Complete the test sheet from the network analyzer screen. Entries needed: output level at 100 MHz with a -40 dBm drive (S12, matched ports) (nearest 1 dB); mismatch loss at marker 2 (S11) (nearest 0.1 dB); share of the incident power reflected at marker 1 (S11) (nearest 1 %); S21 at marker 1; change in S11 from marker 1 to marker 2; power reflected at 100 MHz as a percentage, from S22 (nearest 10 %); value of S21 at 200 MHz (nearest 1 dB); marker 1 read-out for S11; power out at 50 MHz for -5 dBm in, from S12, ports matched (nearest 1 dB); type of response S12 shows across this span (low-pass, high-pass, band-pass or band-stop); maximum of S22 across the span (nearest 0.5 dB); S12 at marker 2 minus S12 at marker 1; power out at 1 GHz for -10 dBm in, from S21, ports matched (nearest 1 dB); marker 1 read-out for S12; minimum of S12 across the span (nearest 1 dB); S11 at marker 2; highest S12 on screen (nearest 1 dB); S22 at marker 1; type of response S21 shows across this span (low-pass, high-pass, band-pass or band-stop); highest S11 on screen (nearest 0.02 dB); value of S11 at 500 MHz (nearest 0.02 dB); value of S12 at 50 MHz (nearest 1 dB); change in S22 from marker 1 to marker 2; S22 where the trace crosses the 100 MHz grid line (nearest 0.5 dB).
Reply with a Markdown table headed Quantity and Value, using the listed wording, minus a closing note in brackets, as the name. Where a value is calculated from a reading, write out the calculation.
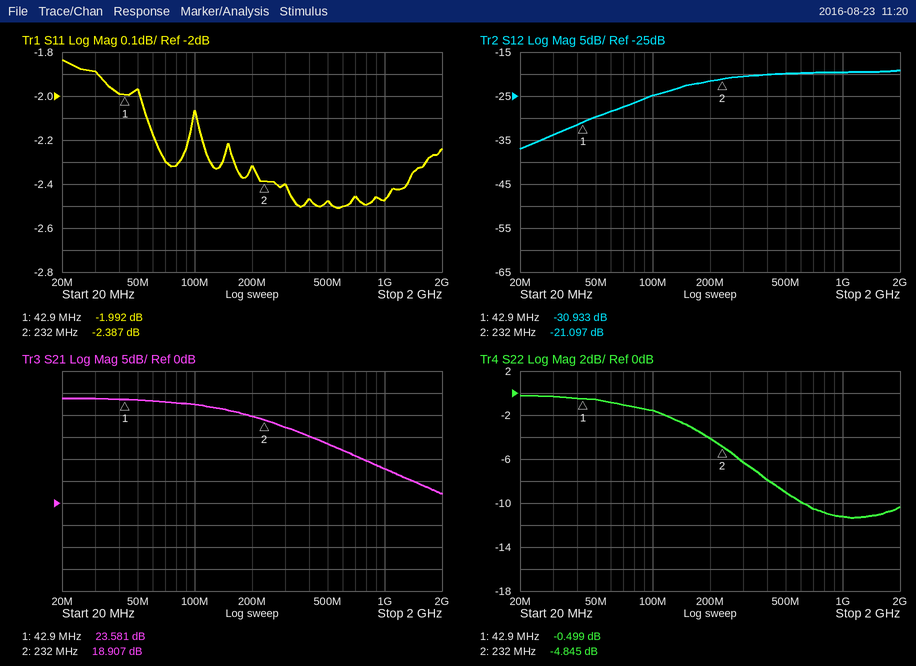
| Quantity | Value |
|---|---|
| output level at 100 MHz with a -40 dBm drive (S12, matched ports) | -40 dBm + (-25 dB) = -65 dBm |
| mismatch loss at marker 2 (S11) | −10 log10(1 − 10^(-2.387/10)) ≈ 3.7 dB |
| share of the incident power reflected at marker 1 (S11) | 10^(-1.992/10) ≈ 63 % |
| S21 at marker 1 | 23.581 dB |
| change in S11 from marker 1 to marker 2 | -2.387 − (-1.992) = -0.395 dB |
| power reflected at 100 MHz as a percentage, from S22 | 10^(-1.5/10) ≈ 70.8 %, so 70 % to the nearest 10 % |
| value of S21 at 200 MHz | 20 dB |
| marker 1 read-out for S11 | -1.992 dB |
| power out at 50 MHz for -5 dBm in, from S12, ports matched | -5 dBm + (-30 dB) = -35 dBm |
| type of response S12 shows across this span | high-pass |
| maximum of S22 across the span | 0.0 dB |
| S12 at marker 2 minus S12 at marker 1 | -21.097 − (-30.933) = 9.836 dB |
| power out at 1 GHz for -10 dBm in, from S21, ports matched | -10 dBm + (8 dB) = -2 dBm |
| marker 1 read-out for S12 | -30.933 dB |
| minimum of S12 across the span | -37 dB |
| S11 at marker 2 | -2.387 dB |
| highest S12 on screen | -19 dB |
| S22 at marker 1 | -0.499 dB |
| type of response S21 shows across this span | low-pass |
| highest S11 on screen | -1.84 dB |
| value of S11 at 500 MHz | -2.48 dB |
| value of S12 at 50 MHz | -30 dB |
| change in S22 from marker 1 to marker 2 | -4.845 − (-0.499) = -4.346 dB |
| S22 where the trace crosses the 100 MHz grid line | -1.5 dB |
